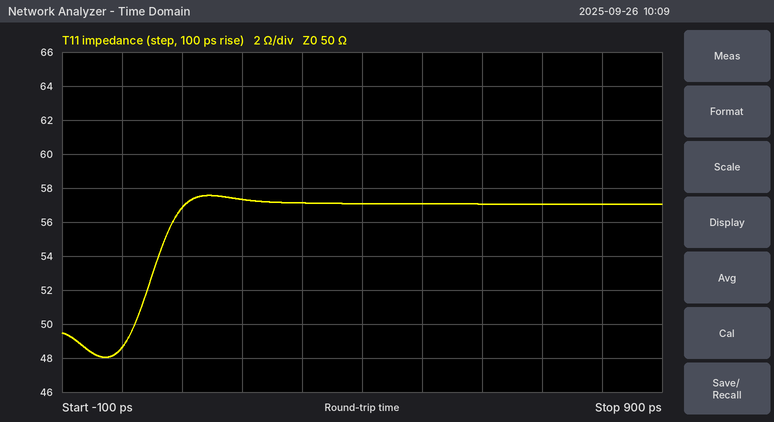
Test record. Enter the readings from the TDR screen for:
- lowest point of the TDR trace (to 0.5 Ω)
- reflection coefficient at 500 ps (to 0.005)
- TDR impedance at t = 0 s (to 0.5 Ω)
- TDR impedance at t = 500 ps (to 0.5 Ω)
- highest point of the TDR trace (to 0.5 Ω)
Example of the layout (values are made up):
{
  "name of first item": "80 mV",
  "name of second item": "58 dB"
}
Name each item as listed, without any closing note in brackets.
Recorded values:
{
  "lowest point of the TDR trace": "48.0 Ω",
  "reflection coefficient at 500 ps": "+0.065",
  "TDR impedance at t = 0 s": "48.5 Ω",
  "TDR impedance at t = 500 ps": "57.0 Ω",
  "highest point of the TDR trace": "57.5 Ω"
}
